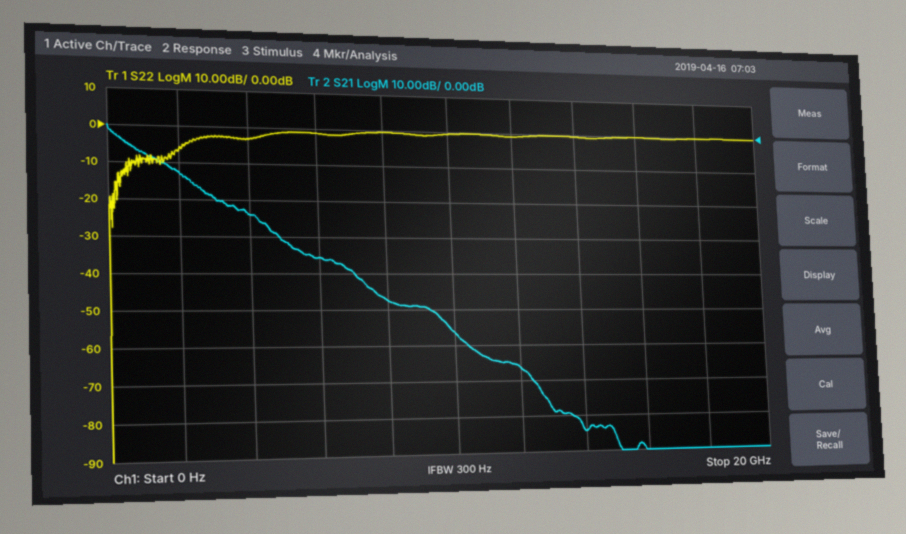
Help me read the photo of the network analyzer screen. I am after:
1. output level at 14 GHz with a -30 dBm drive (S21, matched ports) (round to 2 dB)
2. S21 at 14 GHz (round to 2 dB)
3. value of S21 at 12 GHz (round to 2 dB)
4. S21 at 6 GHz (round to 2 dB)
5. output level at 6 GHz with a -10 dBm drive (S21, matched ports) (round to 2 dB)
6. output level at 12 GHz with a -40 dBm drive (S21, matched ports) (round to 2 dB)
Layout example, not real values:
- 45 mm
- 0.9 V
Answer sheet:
- -114 dBm
- -84 dB
- -66 dB
- -36 dB
- -46 dBm
- -106 dBm
